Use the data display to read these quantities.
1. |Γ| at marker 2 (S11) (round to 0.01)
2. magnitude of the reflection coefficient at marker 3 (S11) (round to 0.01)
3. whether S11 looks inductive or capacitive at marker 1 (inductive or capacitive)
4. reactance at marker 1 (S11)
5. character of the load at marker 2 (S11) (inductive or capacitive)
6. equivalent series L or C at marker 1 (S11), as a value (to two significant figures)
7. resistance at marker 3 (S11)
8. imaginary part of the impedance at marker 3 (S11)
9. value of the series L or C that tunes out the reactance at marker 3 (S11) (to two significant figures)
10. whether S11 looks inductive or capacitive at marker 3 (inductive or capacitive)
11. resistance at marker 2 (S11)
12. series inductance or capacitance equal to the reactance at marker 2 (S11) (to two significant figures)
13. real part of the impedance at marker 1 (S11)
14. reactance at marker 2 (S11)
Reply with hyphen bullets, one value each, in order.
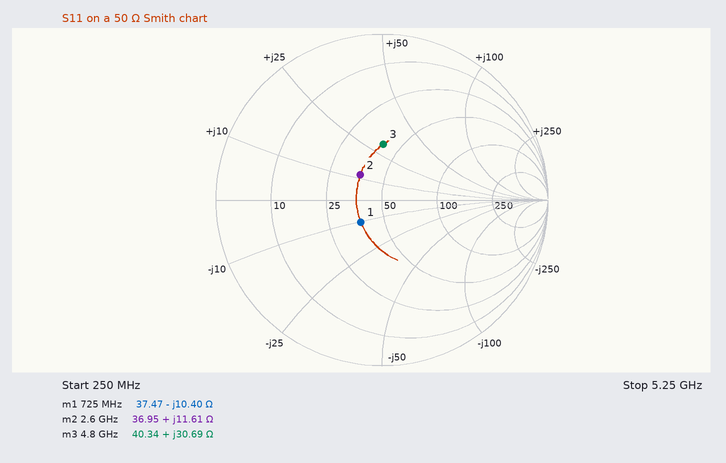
- 0.20
- 0.34
- capacitive
- -10.40 Ω
- inductive
- 21 pF
- 40.34 Ω
- +30.69 Ω
- 1.1 pF
- inductive
- 36.95 Ω
- 710 pH
- 37.47 Ω
- +11.61 Ω
